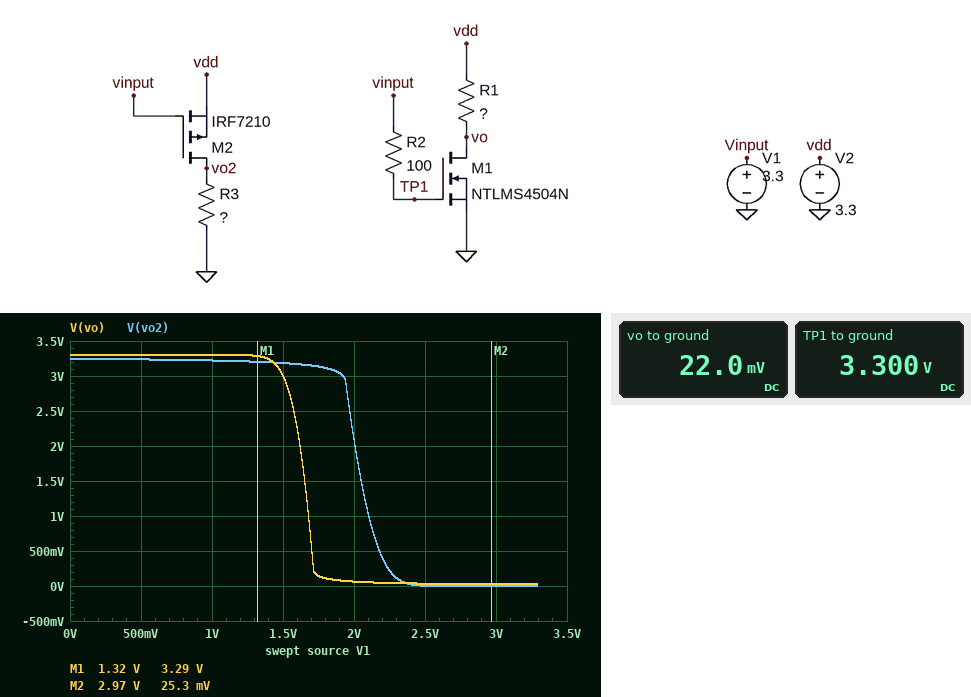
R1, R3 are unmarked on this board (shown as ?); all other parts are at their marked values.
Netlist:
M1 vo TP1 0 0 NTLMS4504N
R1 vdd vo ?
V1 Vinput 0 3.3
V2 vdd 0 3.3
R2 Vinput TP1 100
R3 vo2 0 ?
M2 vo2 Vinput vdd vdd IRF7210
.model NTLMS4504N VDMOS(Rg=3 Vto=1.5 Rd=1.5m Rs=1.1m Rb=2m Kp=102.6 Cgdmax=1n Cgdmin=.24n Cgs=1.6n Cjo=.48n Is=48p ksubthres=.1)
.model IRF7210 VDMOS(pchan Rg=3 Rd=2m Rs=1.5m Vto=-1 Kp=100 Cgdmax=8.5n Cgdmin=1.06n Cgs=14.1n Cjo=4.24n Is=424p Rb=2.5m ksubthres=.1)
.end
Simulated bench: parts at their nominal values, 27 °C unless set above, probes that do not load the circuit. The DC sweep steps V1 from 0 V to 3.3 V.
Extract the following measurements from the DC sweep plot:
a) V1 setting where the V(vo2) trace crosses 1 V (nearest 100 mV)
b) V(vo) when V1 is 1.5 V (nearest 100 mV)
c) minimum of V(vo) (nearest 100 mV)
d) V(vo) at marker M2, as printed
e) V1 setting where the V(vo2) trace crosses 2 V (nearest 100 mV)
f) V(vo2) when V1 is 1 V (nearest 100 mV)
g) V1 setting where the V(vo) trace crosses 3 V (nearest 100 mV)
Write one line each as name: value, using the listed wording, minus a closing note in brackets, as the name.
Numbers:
V1 setting where the V(vo2) trace crosses 1 V: 2.1 V
V(vo) when V1 is 1.5 V: 3.0 V
minimum of V(vo): 0 V
V(vo) at marker M2, as printed: 25.3 mV
V1 setting where the V(vo2) trace crosses 2 V: 2.0 V
V(vo2) when V1 is 1 V: 3.2 V
V1 setting where the V(vo) trace crosses 3 V: 1.5 V
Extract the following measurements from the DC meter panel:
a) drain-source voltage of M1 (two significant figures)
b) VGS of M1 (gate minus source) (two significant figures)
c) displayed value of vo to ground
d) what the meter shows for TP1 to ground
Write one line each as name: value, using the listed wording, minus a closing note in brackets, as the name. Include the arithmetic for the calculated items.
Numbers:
drain-source voltage of M1: 22 mV = 22 mV
VGS of M1 (gate minus source): 3.3 V = 3.3 V
displayed value of vo to ground: 22.0 mV
what the meter shows for TP1 to ground: 3.300 V
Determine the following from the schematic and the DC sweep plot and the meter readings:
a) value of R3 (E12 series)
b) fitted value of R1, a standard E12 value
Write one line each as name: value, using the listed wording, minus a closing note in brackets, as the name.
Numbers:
value of R3: 0.47 Ω
fitted value of R1, a standard E12 value: 1.2 Ω
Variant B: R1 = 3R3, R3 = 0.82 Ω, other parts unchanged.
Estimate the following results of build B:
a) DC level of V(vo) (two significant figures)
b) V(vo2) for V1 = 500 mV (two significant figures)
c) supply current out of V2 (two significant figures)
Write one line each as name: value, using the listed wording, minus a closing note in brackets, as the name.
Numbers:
DC level of V(vo): 8.0 mV
V(vo2) for V1 = 500 mV: 3.3 V
supply current out of V2: 1.0 A
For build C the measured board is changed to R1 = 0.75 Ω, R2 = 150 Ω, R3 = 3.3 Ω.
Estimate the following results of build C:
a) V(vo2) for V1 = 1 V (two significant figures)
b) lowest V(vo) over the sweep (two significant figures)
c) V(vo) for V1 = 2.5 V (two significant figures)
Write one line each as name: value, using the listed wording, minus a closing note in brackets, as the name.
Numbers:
V(vo2) for V1 = 1 V: 3.3 V
lowest V(vo) over the sweep: 35 mV
V(vo) for V1 = 2.5 V: 55 mV
